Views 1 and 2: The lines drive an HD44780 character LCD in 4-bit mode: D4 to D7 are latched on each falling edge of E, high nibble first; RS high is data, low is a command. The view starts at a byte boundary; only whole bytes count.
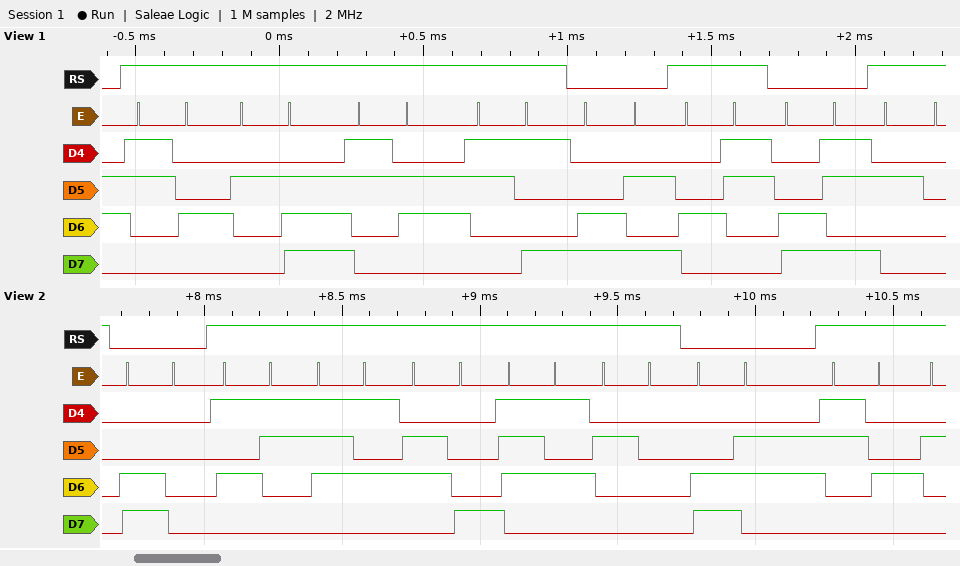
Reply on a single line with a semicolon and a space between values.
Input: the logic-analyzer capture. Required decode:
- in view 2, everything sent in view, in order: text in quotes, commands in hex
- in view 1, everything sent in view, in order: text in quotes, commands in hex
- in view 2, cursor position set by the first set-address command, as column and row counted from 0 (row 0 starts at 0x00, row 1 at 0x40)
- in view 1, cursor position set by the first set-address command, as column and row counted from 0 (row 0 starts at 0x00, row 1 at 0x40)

0xC0 "Suhu " 0xC6 "4"; "4.69" 0xCA "C" 0xCB " "; column 0, row 1; column 10, row 1
